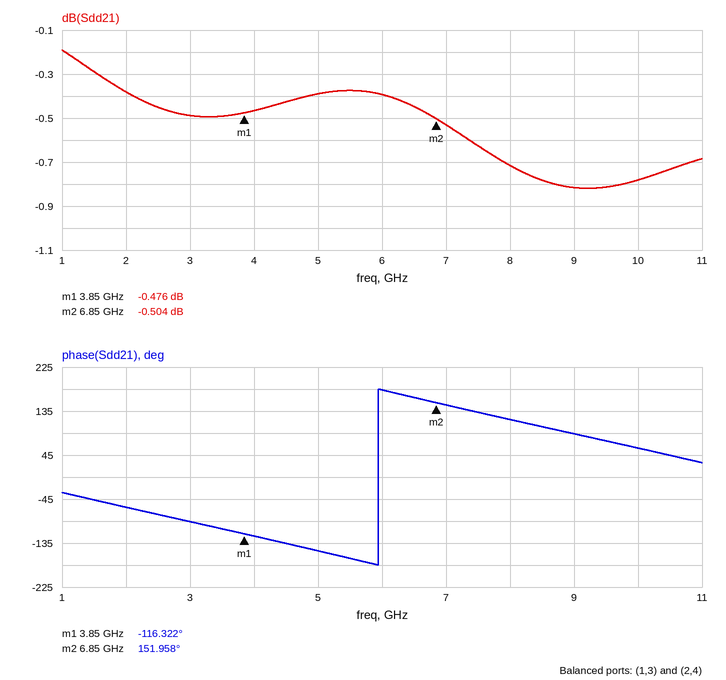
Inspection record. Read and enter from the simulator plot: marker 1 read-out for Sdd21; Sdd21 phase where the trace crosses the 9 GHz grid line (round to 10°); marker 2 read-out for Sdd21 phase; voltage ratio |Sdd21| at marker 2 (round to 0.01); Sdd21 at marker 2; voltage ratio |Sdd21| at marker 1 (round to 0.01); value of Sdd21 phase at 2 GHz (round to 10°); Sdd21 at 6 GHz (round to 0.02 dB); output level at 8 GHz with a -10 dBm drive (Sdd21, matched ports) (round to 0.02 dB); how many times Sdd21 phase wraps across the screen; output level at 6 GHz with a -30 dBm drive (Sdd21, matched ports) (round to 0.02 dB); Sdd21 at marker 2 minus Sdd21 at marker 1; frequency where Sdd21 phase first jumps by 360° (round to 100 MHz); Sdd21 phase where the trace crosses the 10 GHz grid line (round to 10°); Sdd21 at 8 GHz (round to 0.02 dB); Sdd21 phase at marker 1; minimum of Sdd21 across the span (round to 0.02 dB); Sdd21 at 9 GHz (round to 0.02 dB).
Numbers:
-0.476 dB
90°
151.958°
0.94
-0.504 dB
0.95
-60°
-0.40 dB
-10.72 dBm
1
-30.40 dBm
-0.028 dB
5.9 GHz
60°
-0.72 dB
-116.322°
-0.82 dB
-0.82 dB
